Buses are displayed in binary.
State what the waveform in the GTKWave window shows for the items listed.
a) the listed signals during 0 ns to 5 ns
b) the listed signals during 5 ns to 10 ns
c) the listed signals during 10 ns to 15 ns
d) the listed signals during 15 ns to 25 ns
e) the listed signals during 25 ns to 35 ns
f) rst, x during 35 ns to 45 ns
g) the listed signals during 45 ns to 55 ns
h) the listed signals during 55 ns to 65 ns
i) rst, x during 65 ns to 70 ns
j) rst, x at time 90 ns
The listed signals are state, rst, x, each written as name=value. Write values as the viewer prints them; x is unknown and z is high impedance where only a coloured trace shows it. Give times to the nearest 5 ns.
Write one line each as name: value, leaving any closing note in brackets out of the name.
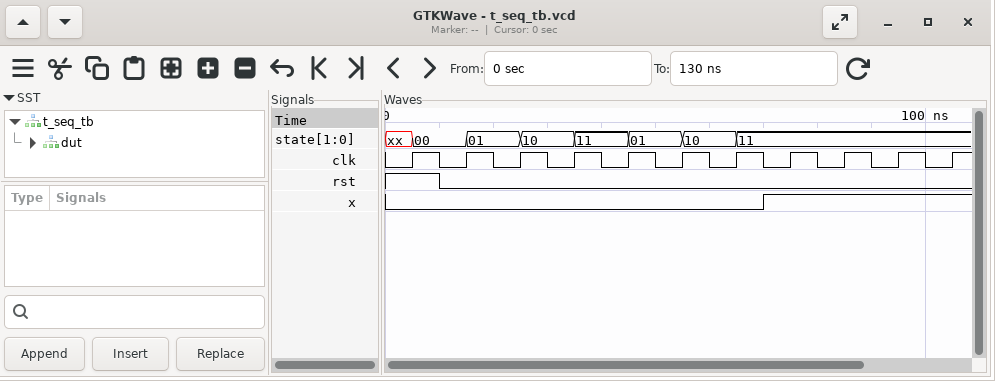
the listed signals during 0 ns to 5 ns: state=xx, rst=1, x=0
the listed signals during 5 ns to 10 ns: state=00, rst=1, x=0
the listed signals during 10 ns to 15 ns: state=00, rst=0, x=0
the listed signals during 15 ns to 25 ns: state=01, rst=0, x=0
the listed signals during 25 ns to 35 ns: state=10, rst=0, x=0
rst, x during 35 ns to 45 ns: rst=0, x=0
the listed signals during 45 ns to 55 ns: state=01, rst=0, x=0
the listed signals during 55 ns to 65 ns: state=10, rst=0, x=0
rst, x during 65 ns to 70 ns: rst=0, x=0
rst, x at time 90 ns: rst=0, x=1
